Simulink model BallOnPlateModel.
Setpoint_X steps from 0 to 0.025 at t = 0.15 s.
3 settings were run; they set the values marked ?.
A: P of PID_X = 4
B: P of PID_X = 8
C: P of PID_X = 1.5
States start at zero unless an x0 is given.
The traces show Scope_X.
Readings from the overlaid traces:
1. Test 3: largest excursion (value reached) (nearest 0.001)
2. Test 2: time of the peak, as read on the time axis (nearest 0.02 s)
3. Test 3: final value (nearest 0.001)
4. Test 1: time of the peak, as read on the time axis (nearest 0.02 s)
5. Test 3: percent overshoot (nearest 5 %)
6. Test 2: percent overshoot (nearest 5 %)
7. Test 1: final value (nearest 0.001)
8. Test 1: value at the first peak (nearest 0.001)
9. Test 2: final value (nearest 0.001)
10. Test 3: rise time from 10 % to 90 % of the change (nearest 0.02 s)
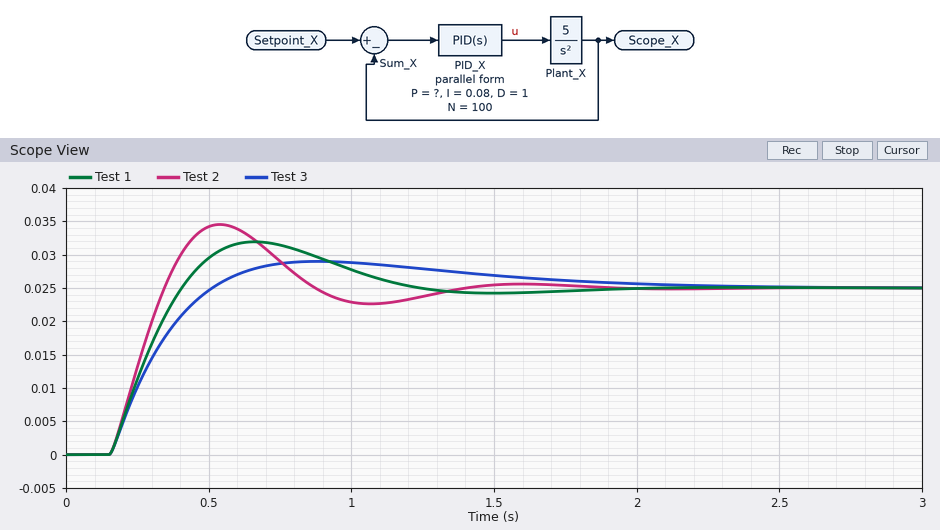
0.029
0.54 s
0.025
0.66 s
15 %
40 %
0.025
0.032
0.025
0.26 s
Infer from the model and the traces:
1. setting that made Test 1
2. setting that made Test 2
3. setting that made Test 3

A
B
C
